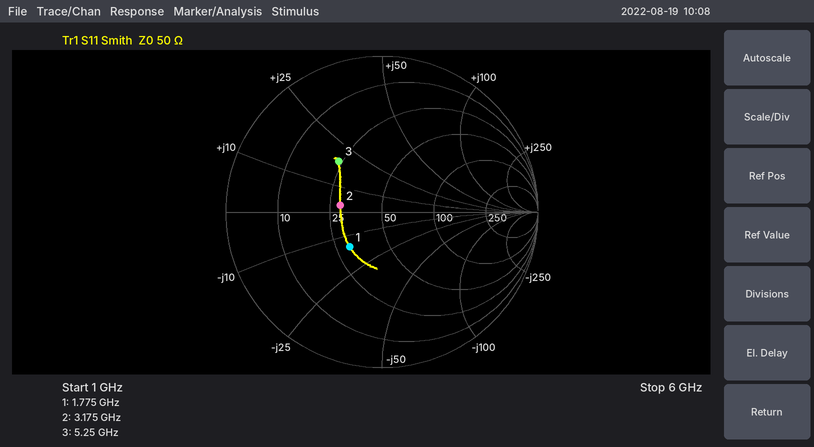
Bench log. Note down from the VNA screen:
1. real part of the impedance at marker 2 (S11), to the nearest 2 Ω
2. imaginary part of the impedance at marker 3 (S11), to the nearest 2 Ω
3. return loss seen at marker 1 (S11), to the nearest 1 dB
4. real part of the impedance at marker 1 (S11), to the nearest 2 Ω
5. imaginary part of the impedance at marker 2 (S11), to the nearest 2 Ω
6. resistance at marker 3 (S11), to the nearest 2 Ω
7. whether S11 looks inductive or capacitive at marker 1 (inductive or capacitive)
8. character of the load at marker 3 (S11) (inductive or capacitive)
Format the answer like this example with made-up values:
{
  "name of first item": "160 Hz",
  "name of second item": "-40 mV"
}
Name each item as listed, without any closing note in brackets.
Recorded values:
{
  "real part of the impedance at marker 2 (S11), to the nearest 2 Ω": "28 Ω",
  "imaginary part of the impedance at marker 3 (S11), to the nearest 2 Ω": "+18 Ω",
  "return loss seen at marker 1 (S11), to the nearest 1 dB": "10 dB",
  "real part of the impedance at marker 1 (S11), to the nearest 2 Ω": "30 Ω",
  "imaginary part of the impedance at marker 2 (S11), to the nearest 2 Ω": "+2 Ω",
  "resistance at marker 3 (S11), to the nearest 2 Ω": "24 Ω",
  "whether S11 looks inductive or capacitive at marker 1": "capacitive",
  "character of the load at marker 3 (S11)": "inductive"
}
